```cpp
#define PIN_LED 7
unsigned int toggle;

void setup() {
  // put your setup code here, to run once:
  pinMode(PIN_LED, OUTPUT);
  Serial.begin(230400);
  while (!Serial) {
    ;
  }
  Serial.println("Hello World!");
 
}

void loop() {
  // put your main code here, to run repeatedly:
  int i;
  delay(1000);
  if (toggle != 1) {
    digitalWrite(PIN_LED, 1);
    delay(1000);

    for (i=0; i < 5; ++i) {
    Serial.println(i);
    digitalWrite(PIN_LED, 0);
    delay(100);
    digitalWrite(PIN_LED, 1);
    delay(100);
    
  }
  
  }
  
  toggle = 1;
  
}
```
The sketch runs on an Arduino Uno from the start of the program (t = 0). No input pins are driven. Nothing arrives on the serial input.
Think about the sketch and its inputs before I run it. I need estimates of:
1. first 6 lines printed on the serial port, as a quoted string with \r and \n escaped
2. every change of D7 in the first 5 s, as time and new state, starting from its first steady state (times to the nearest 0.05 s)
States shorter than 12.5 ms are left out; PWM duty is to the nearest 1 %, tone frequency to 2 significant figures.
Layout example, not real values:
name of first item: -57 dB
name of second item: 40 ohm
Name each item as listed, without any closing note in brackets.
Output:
first 6 lines printed on the serial port, as a quoted string with \r and \n escaped: "Hello World!\r\n0\r\n1\r\n2\r\n3\r\n4\r\n"
every change of D7 in the first 5 s, as time and new state, starting from its first steady state: 0 s low; 1 s high; 2 s low; 2.1 s high; 2.2 s low; 2.3 s high; 2.4 s low; 2.5 s high; 2.6 s low; 2.7 s high; 2.8 s low; 2.9 s high
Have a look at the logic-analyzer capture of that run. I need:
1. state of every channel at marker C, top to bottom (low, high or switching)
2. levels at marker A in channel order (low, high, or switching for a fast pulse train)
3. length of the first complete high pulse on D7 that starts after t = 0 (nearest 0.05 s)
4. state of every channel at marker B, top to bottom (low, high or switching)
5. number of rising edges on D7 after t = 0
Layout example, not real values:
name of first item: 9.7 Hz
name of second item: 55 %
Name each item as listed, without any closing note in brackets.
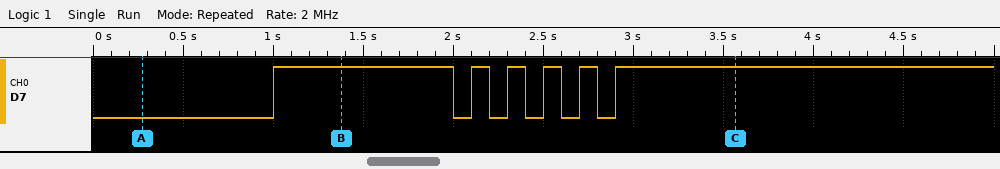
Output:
state of every channel at marker C, top to bottom: D7 high
levels at marker A in channel order: D7 low
length of the first complete high pulse on D7 that starts after t = 0: 1.00 s
state of every channel at marker B, top to bottom: D7 high
number of rising edges on D7 after t = 0: 6
